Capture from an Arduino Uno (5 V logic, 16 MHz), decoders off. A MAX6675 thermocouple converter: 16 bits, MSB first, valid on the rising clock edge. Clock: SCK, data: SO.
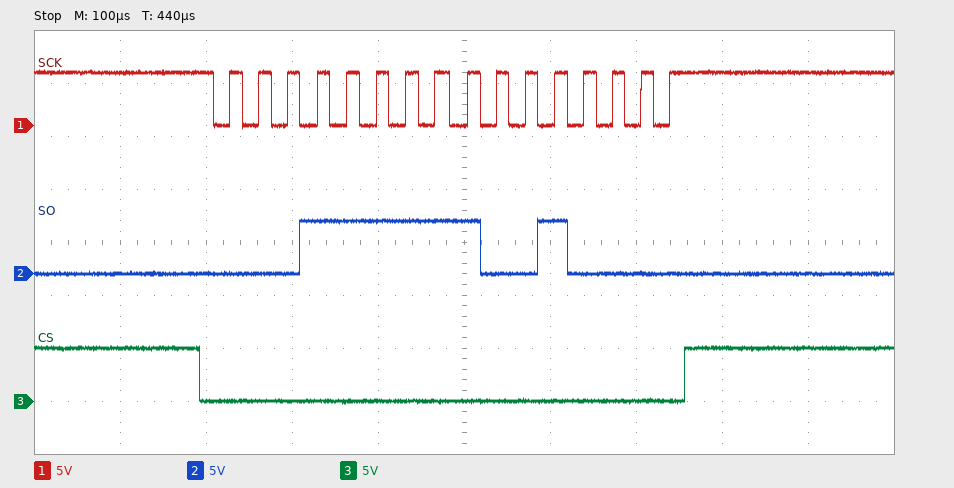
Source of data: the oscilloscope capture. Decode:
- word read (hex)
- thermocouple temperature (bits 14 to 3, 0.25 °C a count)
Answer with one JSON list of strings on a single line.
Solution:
["0x1F90", "252.50 °C"]
